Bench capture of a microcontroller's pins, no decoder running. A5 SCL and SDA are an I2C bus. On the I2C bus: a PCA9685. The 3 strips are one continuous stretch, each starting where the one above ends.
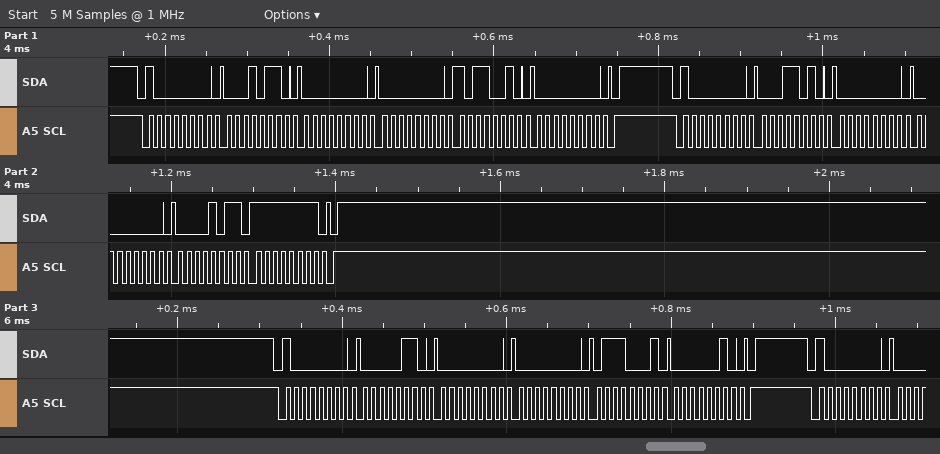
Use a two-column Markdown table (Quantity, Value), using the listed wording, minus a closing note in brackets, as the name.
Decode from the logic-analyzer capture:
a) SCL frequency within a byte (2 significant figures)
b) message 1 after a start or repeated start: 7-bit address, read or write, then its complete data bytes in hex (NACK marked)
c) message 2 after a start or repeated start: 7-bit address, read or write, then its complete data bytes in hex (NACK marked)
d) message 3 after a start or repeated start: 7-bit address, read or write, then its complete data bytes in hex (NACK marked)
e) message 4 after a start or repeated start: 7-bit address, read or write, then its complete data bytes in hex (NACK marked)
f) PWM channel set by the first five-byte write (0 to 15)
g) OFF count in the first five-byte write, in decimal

| Quantity | Value |
|---|---|
| SCL frequency within a byte | 100 kHz |
| message 1 after a start or repeated start: 7-bit address, read or write, then its complete data bytes in hex | 0x40 write: 16 00 00 B2 00 |
| message 2 after a start or repeated start: 7-bit address, read or write, then its complete data bytes in hex | 0x40 write: 1A 00 00 0B FF |
| message 3 after a start or repeated start: 7-bit address, read or write, then its complete data bytes in hex | 0x40 write: 06 00 00 71 02 |
| message 4 after a start or repeated start: 7-bit address, read or write, then its complete data bytes in hex | 0x40 write |
| PWM channel set by the first five-byte write | 4 |
| OFF count in the first five-byte write, in decimal | 178 |
